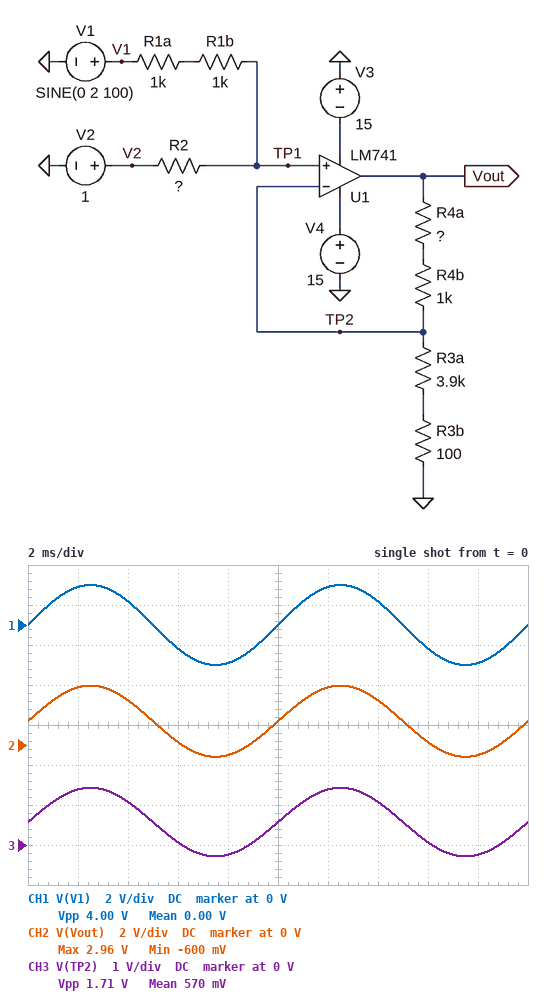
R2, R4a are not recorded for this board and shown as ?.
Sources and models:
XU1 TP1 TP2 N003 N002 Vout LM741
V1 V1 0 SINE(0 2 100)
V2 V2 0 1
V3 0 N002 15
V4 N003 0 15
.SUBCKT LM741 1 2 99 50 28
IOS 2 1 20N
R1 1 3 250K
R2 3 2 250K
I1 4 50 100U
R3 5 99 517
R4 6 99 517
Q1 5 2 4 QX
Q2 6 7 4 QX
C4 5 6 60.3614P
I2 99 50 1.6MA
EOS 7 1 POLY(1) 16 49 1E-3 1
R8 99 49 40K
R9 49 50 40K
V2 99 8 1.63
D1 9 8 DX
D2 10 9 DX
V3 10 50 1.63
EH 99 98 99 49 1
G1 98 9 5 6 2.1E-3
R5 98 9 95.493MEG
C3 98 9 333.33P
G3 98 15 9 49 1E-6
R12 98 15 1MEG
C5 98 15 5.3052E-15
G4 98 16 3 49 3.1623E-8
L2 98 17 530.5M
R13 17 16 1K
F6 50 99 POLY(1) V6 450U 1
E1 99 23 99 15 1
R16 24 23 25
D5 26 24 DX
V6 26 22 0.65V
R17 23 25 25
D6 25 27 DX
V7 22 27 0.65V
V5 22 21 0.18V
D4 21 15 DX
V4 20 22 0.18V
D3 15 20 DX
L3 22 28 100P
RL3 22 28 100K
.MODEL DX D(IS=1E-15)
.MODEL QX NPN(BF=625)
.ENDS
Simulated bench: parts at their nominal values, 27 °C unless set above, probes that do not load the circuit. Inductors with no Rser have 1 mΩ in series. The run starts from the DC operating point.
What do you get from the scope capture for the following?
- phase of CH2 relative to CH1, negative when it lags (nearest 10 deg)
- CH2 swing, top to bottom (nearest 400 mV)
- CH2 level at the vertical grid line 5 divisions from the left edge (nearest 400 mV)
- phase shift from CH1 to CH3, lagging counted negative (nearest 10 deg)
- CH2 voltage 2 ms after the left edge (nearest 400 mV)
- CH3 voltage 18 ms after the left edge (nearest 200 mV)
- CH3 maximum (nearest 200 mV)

0 deg
3.6 V
1.2 V
0 deg
2.8 V
-200 mV
1.4 V
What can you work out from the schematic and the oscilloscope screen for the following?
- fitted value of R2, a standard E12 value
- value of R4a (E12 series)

1.5 kΩ
3.3 kΩ
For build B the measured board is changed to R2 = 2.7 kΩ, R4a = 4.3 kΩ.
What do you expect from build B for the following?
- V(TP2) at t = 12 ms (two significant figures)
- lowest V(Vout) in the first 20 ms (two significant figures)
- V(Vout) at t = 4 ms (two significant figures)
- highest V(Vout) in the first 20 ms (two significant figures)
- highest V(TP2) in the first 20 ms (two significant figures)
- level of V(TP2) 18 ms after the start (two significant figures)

1.5 V
-1.7 V
2.6 V
3.7 V
1.6 V
-670 mV
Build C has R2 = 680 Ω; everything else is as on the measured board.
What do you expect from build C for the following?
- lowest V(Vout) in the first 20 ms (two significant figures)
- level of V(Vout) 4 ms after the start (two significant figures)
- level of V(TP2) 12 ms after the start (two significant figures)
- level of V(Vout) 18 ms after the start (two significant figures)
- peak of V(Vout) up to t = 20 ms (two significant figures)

500 mV
2.2 V
1.2 V
550 mV
2.6 V
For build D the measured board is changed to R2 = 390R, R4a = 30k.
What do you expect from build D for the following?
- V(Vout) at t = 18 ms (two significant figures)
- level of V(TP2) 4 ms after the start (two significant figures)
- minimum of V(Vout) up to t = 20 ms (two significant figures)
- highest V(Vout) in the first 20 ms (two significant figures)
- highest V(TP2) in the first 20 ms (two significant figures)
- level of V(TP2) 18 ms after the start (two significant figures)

4.6 V
1.0 V
4.5 V
10 V
1.2 V
530 mV
